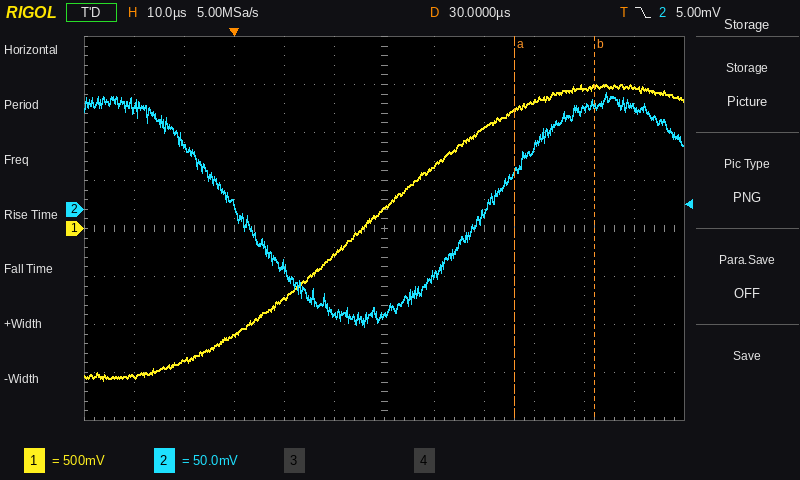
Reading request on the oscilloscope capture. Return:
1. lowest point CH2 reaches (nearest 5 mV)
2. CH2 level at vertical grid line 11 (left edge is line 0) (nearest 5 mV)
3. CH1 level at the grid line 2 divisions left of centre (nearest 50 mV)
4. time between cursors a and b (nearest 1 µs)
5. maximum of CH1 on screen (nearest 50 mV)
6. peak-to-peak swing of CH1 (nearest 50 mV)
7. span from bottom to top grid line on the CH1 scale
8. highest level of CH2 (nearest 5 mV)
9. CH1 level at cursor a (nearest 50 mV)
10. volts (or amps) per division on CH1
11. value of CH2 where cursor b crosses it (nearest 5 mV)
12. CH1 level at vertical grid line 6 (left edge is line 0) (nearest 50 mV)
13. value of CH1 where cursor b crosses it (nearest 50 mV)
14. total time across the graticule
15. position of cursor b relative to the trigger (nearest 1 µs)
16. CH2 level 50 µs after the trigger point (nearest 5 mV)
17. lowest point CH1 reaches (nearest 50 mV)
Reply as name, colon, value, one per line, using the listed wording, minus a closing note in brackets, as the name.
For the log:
lowest point CH2 reaches: -120 mV
CH2 level at vertical grid line 11 (left edge is line 0): 105 mV
CH1 level at the grid line 2 divisions left of centre: -750 mV
time between cursors a and b: 16 µs
maximum of CH1 on screen: 1.50 V
peak-to-peak swing of CH1: 3.10 V
span from bottom to top grid line on the CH1 scale: 4 V
highest level of CH2: 120 mV
CH1 level at cursor a: 1.25 V
volts (or amps) per division on CH1: 500 mV
value of CH2 where cursor b crosses it: 110 mV
CH1 level at vertical grid line 6 (left edge is line 0): 200 mV
value of CH1 where cursor b crosses it: 1.45 V
total time across the graticule: 120 µs
position of cursor b relative to the trigger: +72 µs
CH2 level 50 µs after the trigger point: -5 mV
lowest point CH1 reaches: -1.60 V
